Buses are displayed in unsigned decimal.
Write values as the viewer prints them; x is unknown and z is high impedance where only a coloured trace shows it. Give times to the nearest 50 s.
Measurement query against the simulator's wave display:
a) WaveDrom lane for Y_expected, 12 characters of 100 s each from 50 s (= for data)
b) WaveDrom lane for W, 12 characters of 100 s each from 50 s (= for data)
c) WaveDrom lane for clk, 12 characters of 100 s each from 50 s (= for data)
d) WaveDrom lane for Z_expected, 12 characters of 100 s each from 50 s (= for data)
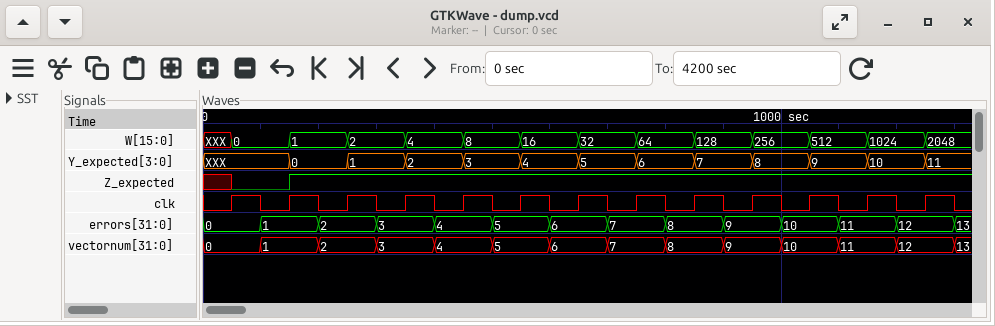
{name: 'Y_expected', wave: 'x===========', data: '0 1 2 3 4 5 6 7 8 9 10'}
{name: 'W', wave: '============', data: '0 1 2 4 8 16 32 64 128 256 512 1024'}
{name: 'clk', wave: 'p...........'}
{name: 'Z_expected', wave: '01..........'}
